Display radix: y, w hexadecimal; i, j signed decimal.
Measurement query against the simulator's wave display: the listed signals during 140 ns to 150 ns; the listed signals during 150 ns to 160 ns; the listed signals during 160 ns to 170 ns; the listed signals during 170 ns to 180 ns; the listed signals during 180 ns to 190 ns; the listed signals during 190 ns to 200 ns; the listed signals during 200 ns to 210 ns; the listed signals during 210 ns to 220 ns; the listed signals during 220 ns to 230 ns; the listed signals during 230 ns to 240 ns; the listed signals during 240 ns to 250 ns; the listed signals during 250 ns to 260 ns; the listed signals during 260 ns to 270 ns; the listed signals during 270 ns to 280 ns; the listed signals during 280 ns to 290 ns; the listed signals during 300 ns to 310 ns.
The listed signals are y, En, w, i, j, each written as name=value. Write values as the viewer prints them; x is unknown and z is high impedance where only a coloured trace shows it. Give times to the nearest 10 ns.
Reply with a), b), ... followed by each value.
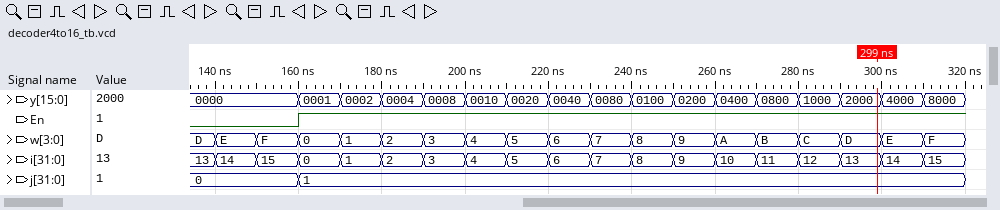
a) y=0000, En=0, w=E, i=14, j=0
b) y=0000, En=0, w=F, i=15, j=0
c) y=0001, En=1, w=0, i=0, j=1
d) y=0002, En=1, w=1, i=1, j=1
e) y=0004, En=1, w=2, i=2, j=1
f) y=0008, En=1, w=3, i=3, j=1
g) y=0010, En=1, w=4, i=4, j=1
h) y=0020, En=1, w=5, i=5, j=1
i) y=0040, En=1, w=6, i=6, j=1
j) y=0080, En=1, w=7, i=7, j=1
k) y=0100, En=1, w=8, i=8, j=1
l) y=0200, En=1, w=9, i=9, j=1
m) y=0400, En=1, w=A, i=10, j=1
n) y=0800, En=1, w=B, i=11, j=1
o) y=1000, En=1, w=C, i=12, j=1
p) y=4000, En=1, w=E, i=14, j=1
